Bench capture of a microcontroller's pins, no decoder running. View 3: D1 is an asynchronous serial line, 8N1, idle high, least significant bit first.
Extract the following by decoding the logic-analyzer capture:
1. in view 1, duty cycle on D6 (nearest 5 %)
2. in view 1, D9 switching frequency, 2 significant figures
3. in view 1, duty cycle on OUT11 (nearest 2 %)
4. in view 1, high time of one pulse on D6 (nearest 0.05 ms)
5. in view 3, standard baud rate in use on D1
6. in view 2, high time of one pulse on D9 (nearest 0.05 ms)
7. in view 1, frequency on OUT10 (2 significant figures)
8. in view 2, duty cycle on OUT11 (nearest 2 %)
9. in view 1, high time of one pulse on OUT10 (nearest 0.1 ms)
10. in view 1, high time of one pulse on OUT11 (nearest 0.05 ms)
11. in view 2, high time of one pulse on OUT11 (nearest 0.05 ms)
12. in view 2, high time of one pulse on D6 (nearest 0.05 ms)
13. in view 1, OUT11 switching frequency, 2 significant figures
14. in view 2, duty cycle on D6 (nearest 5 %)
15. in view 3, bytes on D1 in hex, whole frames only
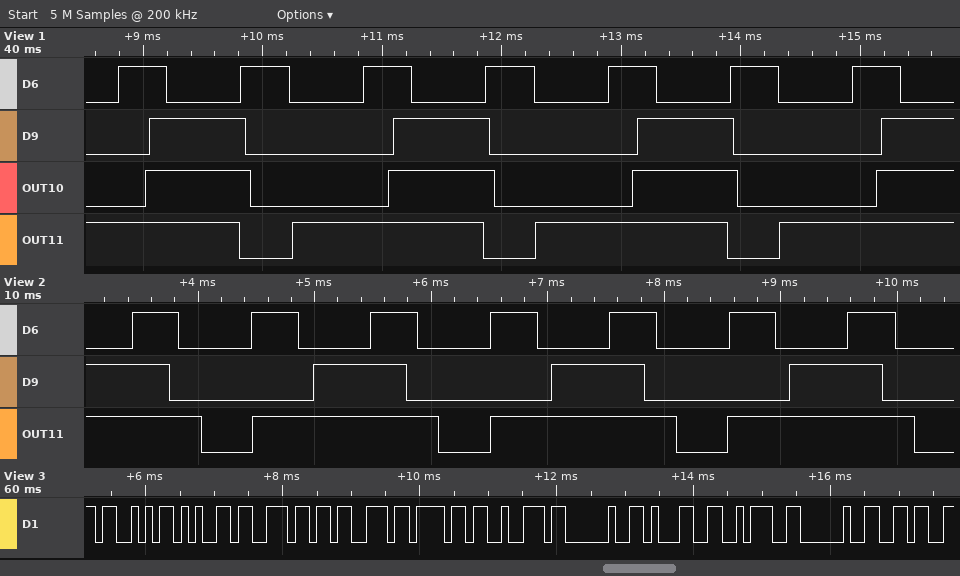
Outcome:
40 %
490 Hz
78 %
0.40 ms
9600 baud
0.80 ms
490 Hz
78 %
0.9 ms
1.60 ms
1.60 ms
0.40 ms
490 Hz
40 %
53 65 6E 73 6F 72 20 31 3A 20 36
